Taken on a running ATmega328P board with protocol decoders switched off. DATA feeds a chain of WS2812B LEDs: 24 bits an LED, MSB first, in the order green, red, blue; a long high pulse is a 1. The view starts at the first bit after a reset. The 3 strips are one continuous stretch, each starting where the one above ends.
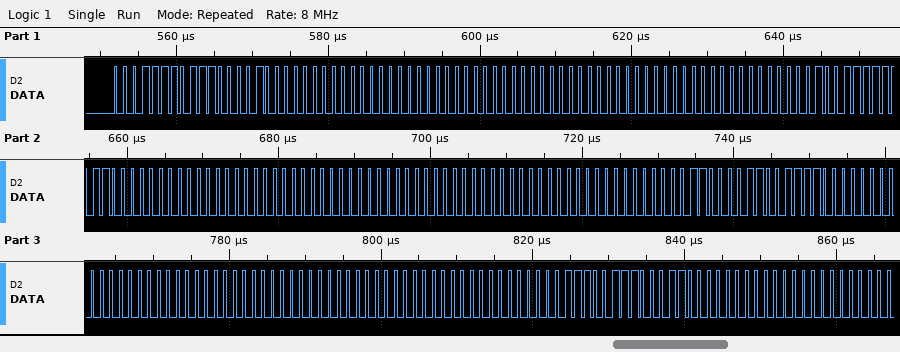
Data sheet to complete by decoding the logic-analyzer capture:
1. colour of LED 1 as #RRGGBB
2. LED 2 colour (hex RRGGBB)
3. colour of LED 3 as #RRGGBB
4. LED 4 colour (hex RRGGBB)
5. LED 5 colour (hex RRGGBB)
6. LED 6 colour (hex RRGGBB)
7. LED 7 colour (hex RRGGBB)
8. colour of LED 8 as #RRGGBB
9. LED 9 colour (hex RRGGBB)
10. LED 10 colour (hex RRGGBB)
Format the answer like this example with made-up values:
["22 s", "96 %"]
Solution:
["#E11E00", "#000000", "#000000", "#D82700", "#000000", "#000000", "#CF3000", "#000000", "#000000", "#C63900"]
